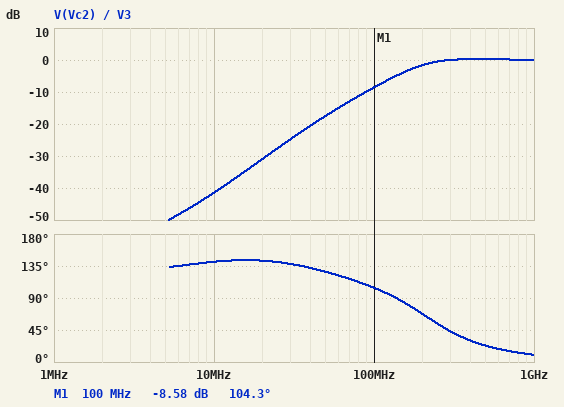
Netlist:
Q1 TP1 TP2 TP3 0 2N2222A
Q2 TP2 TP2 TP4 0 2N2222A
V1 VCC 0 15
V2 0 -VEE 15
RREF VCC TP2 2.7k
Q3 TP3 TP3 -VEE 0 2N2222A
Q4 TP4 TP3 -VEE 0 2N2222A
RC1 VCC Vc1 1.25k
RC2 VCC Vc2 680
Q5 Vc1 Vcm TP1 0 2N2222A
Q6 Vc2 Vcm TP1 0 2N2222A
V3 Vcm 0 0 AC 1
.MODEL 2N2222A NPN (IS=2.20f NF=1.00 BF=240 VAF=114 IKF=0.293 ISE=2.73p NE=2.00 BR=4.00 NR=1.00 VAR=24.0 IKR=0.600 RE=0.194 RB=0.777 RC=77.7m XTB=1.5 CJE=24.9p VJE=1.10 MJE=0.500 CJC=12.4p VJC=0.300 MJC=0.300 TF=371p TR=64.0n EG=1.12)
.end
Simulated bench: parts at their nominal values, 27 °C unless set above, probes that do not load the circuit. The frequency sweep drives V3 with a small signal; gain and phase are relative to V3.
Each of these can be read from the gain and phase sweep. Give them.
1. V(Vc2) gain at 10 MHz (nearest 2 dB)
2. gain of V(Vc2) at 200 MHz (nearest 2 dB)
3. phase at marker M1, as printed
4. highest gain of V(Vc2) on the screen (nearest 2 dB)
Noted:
-42 dB
-2 dB
104.3 deg
0 dB
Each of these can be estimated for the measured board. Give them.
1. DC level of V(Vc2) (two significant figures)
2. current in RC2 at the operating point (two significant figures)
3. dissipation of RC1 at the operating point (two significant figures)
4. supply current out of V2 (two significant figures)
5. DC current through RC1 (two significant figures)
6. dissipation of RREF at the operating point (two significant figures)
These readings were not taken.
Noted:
11 V
5.3 mA
34 mW
21 mA
5.2 mA
300 mW
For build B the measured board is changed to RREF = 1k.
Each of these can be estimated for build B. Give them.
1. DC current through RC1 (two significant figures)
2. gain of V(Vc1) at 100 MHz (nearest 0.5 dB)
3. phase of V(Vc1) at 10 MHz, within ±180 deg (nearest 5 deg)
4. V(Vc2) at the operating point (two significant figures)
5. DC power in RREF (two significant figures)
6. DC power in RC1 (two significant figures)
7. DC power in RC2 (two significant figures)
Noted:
13 mA
0 dB
0 deg
4.6 V
810 mW
200 mW
160 mW
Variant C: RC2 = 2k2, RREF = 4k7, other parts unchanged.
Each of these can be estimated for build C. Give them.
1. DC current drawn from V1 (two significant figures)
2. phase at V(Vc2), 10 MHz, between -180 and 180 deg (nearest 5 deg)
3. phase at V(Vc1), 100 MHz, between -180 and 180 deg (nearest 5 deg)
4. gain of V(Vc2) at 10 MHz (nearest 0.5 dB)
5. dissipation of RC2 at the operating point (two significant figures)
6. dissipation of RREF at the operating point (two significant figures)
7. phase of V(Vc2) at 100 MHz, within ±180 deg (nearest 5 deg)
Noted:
12 mA
75 deg
85 deg
-23.0 dB
20 mW
170 mW
70 deg
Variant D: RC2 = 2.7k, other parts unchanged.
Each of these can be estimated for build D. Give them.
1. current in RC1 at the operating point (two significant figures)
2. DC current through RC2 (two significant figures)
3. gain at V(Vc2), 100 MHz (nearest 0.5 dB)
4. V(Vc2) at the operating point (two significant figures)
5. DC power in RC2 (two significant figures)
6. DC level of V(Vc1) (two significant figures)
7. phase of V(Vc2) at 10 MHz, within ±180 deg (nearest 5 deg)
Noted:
5.4 mA
5.1 mA
-5.0 dB
1.2 V
70 mW
8.2 V
40 deg
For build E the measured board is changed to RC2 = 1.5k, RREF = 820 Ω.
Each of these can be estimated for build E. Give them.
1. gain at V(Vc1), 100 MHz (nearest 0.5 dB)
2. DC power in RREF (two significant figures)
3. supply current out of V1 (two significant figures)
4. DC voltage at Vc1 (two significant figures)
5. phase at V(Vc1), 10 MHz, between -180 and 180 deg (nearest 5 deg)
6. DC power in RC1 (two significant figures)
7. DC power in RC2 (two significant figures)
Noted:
0 dB
980 mW
58 mA
-780 mV
0 deg
200 mW
170 mW
